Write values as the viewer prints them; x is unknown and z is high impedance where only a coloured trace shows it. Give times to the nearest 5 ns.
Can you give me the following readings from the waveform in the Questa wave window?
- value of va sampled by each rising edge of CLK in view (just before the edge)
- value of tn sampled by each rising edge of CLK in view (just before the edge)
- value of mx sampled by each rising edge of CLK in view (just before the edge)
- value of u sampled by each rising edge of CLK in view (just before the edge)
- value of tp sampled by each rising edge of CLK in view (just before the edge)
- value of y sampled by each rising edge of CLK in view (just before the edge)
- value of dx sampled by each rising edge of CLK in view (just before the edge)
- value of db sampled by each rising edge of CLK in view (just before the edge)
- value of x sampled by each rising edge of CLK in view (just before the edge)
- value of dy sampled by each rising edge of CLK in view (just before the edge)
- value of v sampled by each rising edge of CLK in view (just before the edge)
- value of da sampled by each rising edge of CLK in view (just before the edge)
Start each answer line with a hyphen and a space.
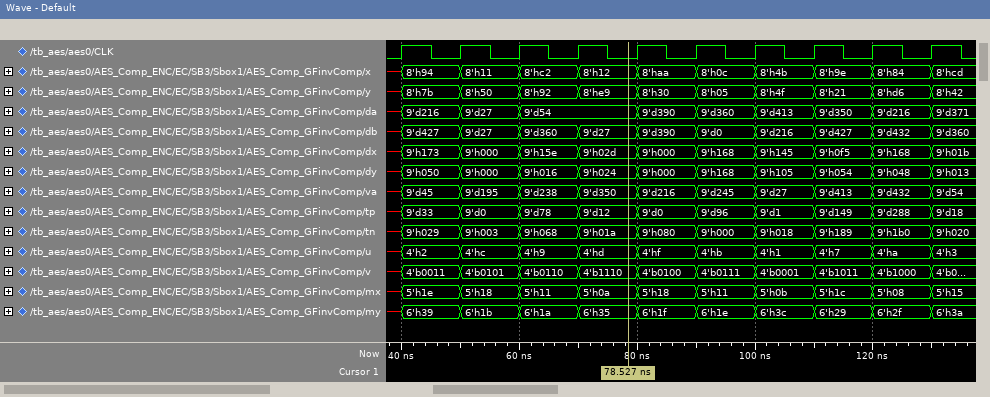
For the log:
- x, 9'd45, 9'd195, 9'd238, 9'd350, 9'd216, 9'd245, 9'd27, 9'd413, 9'd432
- x, 9'h029, 9'h003, 9'h068, 9'h01a, 9'h080, 9'h000, 9'h018, 9'h189, 9'h1b0
- x, 5'h1e, 5'h18, 5'h11, 5'h0a, 5'h18, 5'h11, 5'h0b, 5'h1c, 5'h08
- x, 4'h2, 4'hc, 4'h9, 4'hd, 4'hf, 4'hb, 4'h1, 4'h7, 4'ha
- x, 9'd33, 9'd0, 9'd78, 9'd12, 9'd0, 9'd96, 9'd1, 9'd149, 9'd288
- x, 8'h7b, 8'h50, 8'h92, 8'he9, 8'h30, 8'h05, 8'h4f, 8'h21, 8'hd6
- x, 9'h173, 9'h000, 9'h15e, 9'h02d, 9'h000, 9'h168, 9'h145, 9'h0f5, 9'h168
- x, 9'd427, 9'd27, 9'd360, 9'd27, 9'd390, 9'd0, 9'd216, 9'd427, 9'd432
- x, 8'h94, 8'h11, 8'hc2, 8'h12, 8'haa, 8'h0c, 8'h4b, 8'h9e, 8'h84
- x, 9'h050, 9'h000, 9'h016, 9'h024, 9'h000, 9'h168, 9'h105, 9'h054, 9'h048
- x, 4'b0011, 4'b0101, 4'b0110, 4'b1110, 4'b0100, 4'b0111, 4'b0001, 4'b1011, 4'b1000
- x, 9'd216, 9'd27, 9'd54, 9'd54, 9'd390, 9'd360, 9'd413, 9'd350, 9'd216
